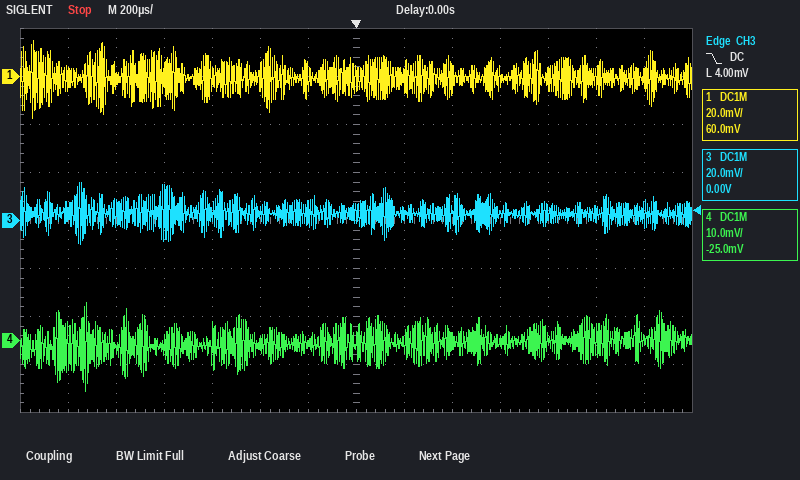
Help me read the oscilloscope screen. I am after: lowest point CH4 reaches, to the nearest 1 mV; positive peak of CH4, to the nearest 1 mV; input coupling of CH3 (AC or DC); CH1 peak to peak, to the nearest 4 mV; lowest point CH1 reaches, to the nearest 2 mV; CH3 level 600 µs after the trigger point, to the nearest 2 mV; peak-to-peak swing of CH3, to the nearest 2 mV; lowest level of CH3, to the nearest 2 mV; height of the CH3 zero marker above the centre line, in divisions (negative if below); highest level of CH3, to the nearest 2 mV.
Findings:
-11 mV
8 mV
DC
32 mV
-18 mV
2 mV
26 mV
-10 mV
0.0 div
16 mV
